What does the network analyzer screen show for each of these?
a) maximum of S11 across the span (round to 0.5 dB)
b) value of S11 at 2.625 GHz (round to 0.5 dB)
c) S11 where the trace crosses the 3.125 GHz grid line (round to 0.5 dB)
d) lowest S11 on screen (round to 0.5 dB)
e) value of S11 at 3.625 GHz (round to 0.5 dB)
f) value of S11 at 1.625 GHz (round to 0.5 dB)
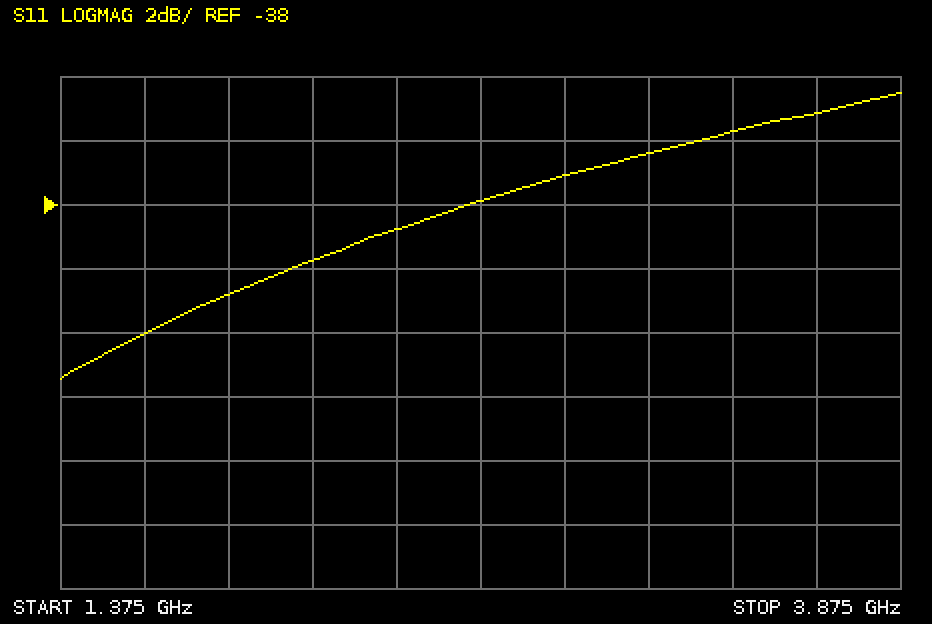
-34.5 dB
-38.0 dB
-36.5 dB
-43.5 dB
-35.0 dB
-42.0 dB
